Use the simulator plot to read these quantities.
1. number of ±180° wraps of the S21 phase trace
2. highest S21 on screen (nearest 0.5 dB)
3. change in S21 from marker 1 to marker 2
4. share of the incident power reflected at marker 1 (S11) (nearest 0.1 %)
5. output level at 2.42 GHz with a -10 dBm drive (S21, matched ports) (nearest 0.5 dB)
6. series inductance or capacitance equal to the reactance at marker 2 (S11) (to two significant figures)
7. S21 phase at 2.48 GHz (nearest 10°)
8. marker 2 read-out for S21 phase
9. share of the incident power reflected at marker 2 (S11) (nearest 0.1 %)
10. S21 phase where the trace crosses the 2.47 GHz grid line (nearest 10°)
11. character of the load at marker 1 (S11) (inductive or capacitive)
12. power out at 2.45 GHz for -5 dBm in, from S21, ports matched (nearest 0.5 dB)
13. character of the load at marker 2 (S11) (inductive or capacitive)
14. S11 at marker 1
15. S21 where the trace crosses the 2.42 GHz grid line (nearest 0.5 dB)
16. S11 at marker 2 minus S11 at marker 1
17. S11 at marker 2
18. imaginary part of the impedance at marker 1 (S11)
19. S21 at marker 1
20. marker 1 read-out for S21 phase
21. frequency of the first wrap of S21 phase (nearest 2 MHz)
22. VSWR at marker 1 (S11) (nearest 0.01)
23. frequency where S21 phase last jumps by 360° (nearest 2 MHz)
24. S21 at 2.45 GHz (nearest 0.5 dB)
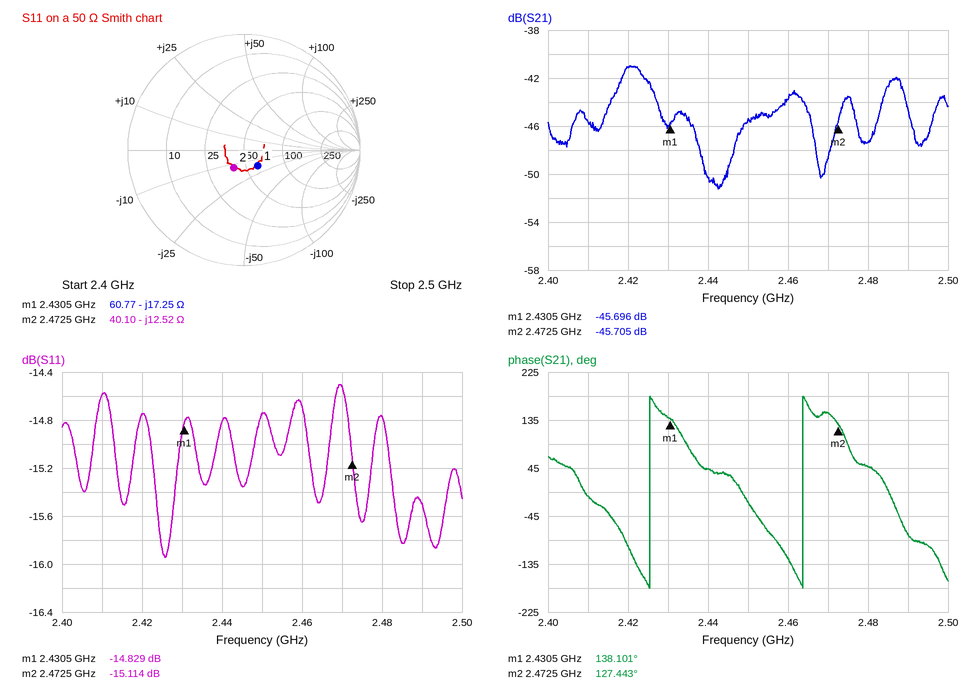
2
-41.0 dB
-0.009 dB
3.3 %
-51.0 dBm
5.1 pF
50°
127.443°
3.1 %
150°
capacitive
-50.5 dBm
capacitive
-14.829 dB
-41.0 dB
-0.285 dB
-15.114 dB
-17.25 Ω
-45.696 dB
138.101°
2.426 GHz
1.44
2.464 GHz
-45.5 dB
